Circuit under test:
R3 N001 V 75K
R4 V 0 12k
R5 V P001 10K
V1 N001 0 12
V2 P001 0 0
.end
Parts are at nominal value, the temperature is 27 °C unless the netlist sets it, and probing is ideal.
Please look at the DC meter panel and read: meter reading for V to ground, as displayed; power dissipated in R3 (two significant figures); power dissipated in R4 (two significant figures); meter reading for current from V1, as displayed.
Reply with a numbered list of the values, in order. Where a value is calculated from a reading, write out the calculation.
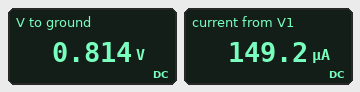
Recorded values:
1. 0.814 V
2. (12 V - 814 mV)^2 / 75 kΩ = 1.7 mW
3. (814 mV)^2 / 12 kΩ = 55 µW
4. 149.2 µA
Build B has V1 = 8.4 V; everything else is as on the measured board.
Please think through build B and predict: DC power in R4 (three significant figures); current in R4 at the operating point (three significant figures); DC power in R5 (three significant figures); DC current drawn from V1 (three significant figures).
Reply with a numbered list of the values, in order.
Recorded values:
1. 27.0 µW
2. 47.5 µA
3. 32.4 µW
4. 104 µA
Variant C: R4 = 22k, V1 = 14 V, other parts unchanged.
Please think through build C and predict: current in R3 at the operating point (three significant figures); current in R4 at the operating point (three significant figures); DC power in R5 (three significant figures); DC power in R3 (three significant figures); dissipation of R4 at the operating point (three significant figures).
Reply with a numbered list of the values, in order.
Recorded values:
1. 171 µA
2. 53.4 µA
3. 138 µW
4. 2.19 mW
5. 62.8 µW
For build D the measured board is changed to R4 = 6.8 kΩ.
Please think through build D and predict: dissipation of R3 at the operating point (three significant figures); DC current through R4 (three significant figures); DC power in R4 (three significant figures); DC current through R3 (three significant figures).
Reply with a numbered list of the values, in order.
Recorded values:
1. 1.73 mW
2. 90.4 µA
3. 55.5 µW
4. 152 µA
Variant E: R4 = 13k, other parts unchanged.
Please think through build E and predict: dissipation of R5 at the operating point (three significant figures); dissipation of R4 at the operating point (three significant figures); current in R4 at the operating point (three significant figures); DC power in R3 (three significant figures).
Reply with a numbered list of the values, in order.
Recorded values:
1. 70.7 µW
2. 54.4 µW
3. 64.7 µA
4. 1.66 mW
